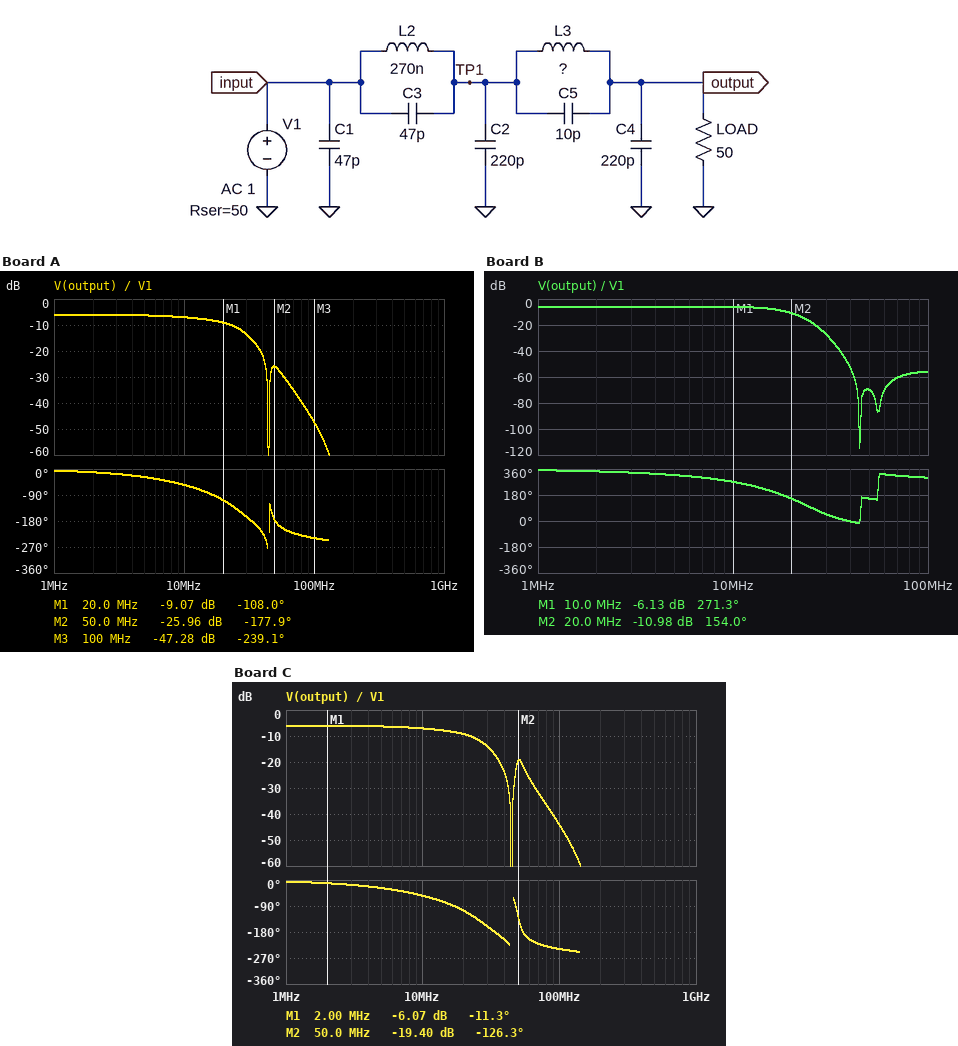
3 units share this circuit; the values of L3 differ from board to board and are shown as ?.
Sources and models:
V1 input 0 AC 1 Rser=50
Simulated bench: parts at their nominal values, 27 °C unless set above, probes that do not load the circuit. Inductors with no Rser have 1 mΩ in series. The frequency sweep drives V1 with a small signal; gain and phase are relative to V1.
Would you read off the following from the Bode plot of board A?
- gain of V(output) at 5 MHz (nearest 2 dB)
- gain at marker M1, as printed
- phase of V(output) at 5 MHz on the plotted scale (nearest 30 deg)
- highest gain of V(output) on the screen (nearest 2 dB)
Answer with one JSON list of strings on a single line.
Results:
["-6 dB", "-9.07 dB", "-30 deg", "-6 dB"]
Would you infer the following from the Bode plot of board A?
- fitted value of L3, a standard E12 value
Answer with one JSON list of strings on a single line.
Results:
["100 nH"]
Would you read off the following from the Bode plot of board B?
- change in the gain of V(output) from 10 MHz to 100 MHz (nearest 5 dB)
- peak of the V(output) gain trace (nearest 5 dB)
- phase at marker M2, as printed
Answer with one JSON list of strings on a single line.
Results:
["-50 dB", "-5 dB", "154.0 deg"]
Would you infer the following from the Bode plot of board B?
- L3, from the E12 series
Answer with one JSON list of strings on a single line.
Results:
["820 nH"]
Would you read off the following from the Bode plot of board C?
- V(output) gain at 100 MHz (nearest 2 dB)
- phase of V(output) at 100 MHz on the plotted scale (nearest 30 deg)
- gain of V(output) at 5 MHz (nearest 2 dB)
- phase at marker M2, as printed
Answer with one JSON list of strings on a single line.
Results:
["-44 dB", "-240 deg", "-6 dB", "-126.3 deg"]
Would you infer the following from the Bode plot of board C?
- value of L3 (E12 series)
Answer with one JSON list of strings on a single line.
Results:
["82 nH"]
